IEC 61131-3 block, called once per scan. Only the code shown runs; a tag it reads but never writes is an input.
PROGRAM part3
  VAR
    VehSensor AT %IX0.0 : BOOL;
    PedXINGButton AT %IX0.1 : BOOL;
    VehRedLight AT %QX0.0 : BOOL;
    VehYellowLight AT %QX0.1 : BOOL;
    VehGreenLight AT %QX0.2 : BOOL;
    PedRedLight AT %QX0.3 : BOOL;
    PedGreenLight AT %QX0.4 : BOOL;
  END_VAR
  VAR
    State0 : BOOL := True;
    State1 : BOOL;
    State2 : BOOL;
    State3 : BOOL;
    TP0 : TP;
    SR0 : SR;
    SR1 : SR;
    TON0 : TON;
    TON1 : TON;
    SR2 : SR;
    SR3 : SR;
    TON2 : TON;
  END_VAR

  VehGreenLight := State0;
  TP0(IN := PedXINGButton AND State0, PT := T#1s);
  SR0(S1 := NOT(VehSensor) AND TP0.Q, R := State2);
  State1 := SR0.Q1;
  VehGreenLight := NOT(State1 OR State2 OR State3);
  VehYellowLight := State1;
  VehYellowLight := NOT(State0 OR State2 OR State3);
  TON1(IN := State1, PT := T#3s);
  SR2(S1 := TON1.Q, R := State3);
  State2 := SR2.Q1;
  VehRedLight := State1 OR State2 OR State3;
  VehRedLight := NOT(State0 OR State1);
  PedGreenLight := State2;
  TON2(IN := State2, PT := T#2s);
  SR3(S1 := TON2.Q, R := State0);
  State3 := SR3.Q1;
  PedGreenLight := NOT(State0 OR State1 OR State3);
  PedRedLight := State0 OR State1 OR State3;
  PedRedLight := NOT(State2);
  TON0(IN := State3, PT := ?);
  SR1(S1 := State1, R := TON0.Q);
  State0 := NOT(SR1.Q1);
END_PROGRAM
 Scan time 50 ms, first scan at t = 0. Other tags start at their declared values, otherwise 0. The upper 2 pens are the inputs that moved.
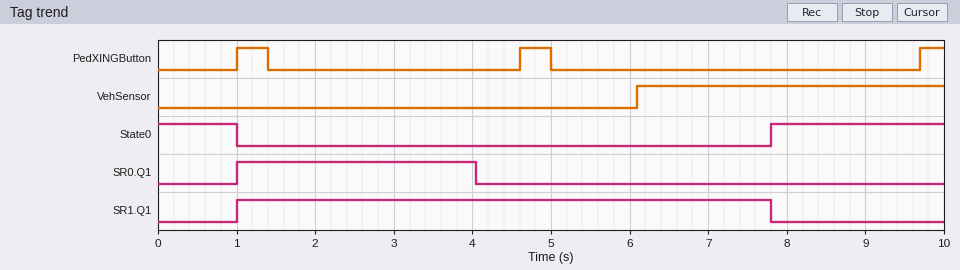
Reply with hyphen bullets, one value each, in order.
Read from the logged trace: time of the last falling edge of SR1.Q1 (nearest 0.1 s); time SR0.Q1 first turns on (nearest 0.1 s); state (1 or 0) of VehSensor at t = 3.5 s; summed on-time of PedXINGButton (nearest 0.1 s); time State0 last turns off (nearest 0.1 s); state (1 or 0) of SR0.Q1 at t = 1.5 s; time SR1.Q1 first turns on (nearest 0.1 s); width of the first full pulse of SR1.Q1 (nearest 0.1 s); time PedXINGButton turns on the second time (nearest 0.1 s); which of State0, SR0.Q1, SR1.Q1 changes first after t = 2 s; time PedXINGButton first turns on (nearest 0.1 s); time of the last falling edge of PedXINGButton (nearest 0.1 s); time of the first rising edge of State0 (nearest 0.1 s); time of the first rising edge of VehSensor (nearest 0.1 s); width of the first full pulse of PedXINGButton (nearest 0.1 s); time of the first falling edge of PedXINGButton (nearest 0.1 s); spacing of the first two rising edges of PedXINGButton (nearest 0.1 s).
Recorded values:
- 7.8 s
- 1.0 s
- 0
- 1.1 s
- 1.0 s
- 1
- 1.0 s
- 6.8 s
- 4.6 s
- SR0.Q1
- 1.0 s
- 5.0 s
- 7.8 s
- 6.1 s
- 0.4 s
- 1.4 s
- 3.6 s
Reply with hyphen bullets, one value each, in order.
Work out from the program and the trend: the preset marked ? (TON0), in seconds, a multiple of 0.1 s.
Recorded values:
- 1.8 s
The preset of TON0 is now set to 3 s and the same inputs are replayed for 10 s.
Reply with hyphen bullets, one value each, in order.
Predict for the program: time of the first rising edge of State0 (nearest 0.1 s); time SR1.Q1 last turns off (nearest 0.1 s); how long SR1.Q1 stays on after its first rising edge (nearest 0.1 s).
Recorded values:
- 9.0 s
- 9.0 s
- 8.0 s
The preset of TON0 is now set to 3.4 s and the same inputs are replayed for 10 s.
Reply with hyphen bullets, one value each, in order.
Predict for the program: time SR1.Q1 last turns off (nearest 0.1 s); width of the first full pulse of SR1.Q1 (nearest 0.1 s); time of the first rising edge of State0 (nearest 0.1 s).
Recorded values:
- 9.4 s
- 8.4 s
- 9.4 s
